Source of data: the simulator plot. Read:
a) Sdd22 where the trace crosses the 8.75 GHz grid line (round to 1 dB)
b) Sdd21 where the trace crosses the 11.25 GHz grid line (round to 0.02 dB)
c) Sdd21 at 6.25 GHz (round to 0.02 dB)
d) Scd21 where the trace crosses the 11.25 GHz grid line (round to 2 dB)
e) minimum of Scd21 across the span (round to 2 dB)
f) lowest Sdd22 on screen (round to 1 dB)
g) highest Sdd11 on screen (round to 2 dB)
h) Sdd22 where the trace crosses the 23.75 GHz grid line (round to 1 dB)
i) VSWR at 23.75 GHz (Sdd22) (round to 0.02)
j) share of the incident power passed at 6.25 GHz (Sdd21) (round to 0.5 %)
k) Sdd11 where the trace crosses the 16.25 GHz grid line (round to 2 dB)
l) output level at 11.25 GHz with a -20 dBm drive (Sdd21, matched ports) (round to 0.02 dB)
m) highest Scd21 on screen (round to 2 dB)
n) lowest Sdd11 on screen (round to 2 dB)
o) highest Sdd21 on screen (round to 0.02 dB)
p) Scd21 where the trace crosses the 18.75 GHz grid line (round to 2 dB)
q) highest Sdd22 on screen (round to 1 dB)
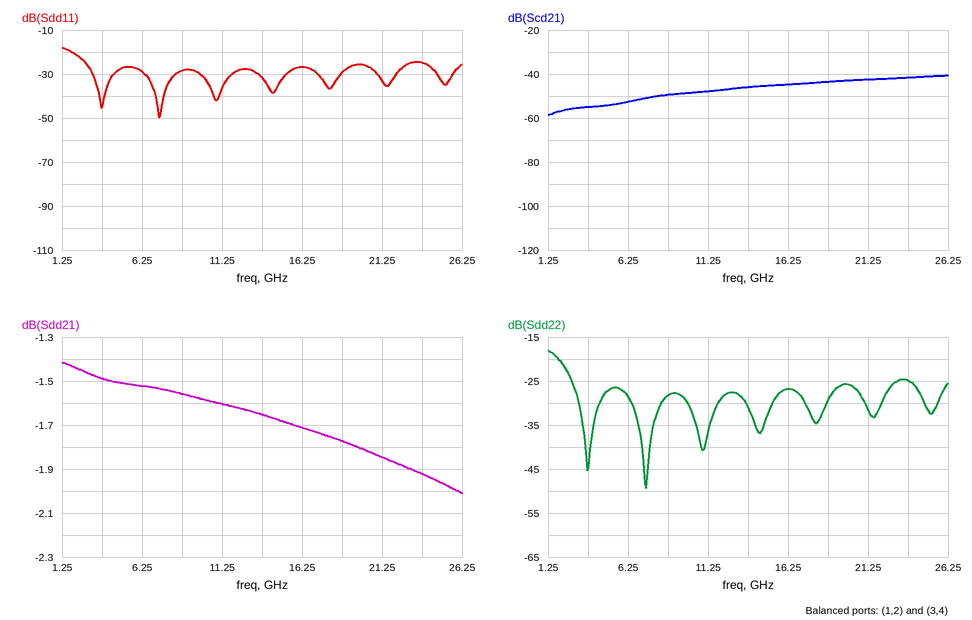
-28 dB
-1.60 dB
-1.52 dB
-48 dB
-58 dB
-49 dB
-18 dB
-25 dB
1.12
70.5 %
-26 dB
-21.60 dBm
-40 dB
-50 dB
-1.42 dB
-44 dB
-18 dB
